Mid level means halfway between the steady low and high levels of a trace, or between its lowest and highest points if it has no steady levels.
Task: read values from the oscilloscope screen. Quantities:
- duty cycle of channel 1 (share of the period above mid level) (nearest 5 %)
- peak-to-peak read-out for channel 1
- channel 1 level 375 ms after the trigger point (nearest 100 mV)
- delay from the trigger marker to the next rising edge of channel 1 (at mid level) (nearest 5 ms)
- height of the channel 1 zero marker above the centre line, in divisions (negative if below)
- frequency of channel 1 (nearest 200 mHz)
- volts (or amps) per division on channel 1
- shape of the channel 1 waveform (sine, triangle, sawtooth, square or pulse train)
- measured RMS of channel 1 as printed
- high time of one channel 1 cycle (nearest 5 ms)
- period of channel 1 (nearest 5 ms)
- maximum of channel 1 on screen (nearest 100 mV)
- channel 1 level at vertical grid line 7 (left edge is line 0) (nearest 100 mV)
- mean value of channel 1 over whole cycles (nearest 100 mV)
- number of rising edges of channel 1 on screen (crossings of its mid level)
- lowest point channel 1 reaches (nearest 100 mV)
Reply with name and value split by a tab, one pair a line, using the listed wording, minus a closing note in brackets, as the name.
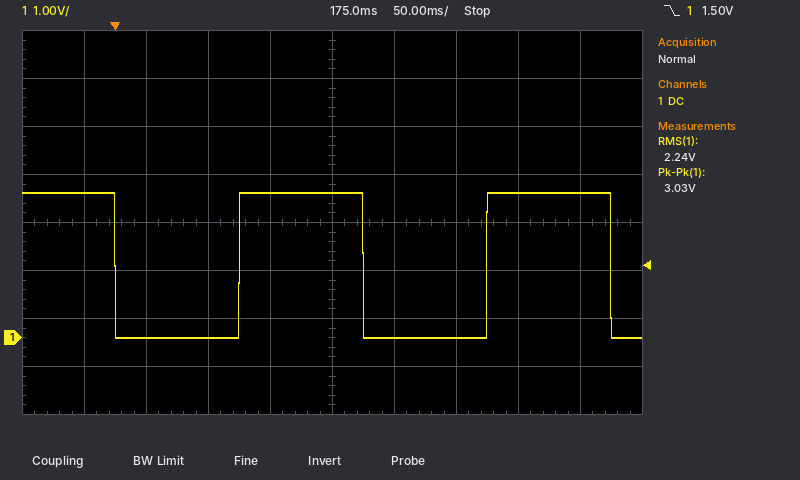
duty cycle of channel 1 (share of the period above mid level)	50 %
peak-to-peak read-out for channel 1	3.03 V
channel 1 level 375 ms after the trigger point	3.0 V
delay from the trigger marker to the next rising edge of channel 1 (at mid level)	100 ms
height of the channel 1 zero marker above the centre line, in divisions	-2.4 div
frequency of channel 1	5.0 Hz
volts (or amps) per division on channel 1	1 V
shape of the channel 1 waveform	square
measured RMS of channel 1 as printed	2.24 V
high time of one channel 1 cycle	100 ms
period of channel 1	200 ms
maximum of channel 1 on screen	3.0 V
channel 1 level at vertical grid line 7 (left edge is line 0)	0.0 V
mean value of channel 1 over whole cycles	1.5 V
number of rising edges of channel 1 on screen	2
lowest point channel 1 reaches	0.0 V
